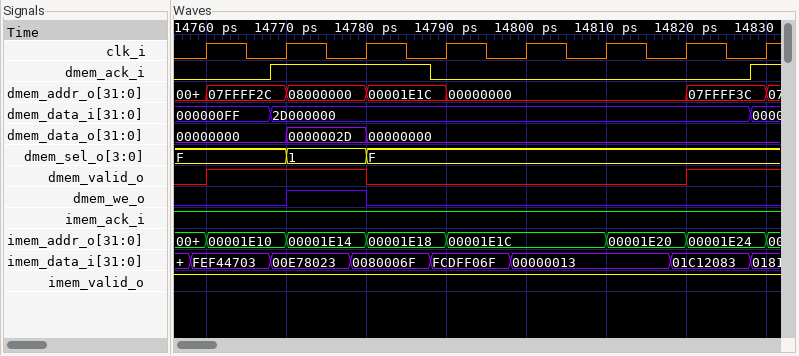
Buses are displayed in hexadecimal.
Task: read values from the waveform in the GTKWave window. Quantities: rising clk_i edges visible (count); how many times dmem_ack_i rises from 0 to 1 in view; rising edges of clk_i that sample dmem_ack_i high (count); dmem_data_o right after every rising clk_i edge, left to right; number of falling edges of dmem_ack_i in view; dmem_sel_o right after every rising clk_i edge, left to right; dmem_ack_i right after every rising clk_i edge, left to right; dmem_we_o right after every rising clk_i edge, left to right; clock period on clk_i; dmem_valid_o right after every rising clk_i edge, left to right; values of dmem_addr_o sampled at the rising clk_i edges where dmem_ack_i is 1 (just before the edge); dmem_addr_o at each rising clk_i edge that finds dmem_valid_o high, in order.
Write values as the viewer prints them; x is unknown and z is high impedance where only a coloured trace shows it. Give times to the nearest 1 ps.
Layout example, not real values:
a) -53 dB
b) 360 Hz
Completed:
a) 8
b) 2
c) 3
d) 00000000, 0000002D, 00000000, 00000000, 00000000, 00000000, 00000000, 00000000
e) 1
f) F, 1, F, F, F, F, F, F
g) 0 1 1 0 0 0 0 1
h) 0 1 0 0 0 0 0 0
i) 10 ps
j) 1 1 0 0 0 0 1 1
k) 07FFFF2C, 08000000, 07FFFF3C
l) 07FFFF2C, 08000000, 07FFFF3C
